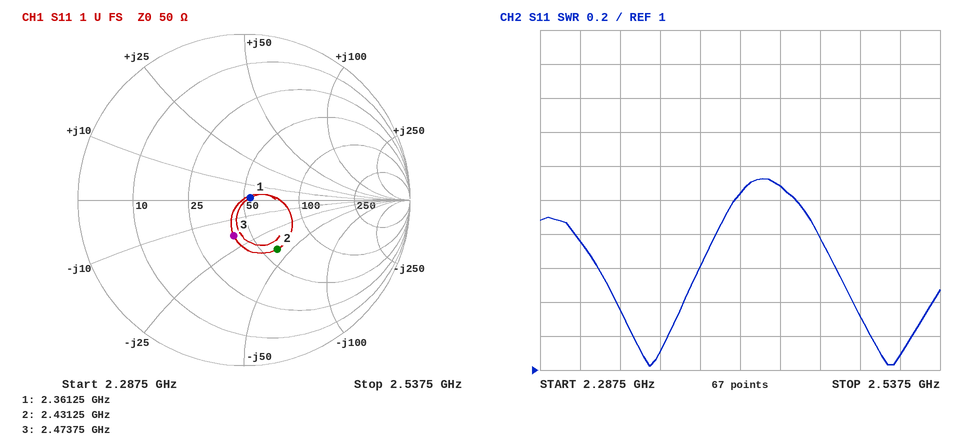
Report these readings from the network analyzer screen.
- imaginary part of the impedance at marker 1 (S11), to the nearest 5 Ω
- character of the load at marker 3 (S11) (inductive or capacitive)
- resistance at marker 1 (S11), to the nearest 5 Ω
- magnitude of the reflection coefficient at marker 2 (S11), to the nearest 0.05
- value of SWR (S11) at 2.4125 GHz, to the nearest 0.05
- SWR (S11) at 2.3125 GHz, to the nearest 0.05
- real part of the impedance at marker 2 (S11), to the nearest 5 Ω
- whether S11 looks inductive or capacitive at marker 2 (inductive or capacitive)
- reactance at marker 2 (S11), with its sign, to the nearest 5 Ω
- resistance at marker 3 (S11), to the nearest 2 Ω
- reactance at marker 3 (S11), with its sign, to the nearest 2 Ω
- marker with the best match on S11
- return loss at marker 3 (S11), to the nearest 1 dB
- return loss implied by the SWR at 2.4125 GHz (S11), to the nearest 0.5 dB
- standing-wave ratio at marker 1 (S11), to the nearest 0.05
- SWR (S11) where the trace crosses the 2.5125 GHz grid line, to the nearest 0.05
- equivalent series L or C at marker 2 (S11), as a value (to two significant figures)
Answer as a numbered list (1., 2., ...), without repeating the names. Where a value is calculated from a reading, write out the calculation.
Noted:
1. 0 Ω
2. capacitive
3. 55 Ω
4. 0.35
5. 2.05
6. 1.75
7. 60 Ω
8. capacitive
9. -40 Ω
10. 40 Ω
11. -18 Ω
12. marker 1
13. 13 dB
14. −20 log10((2.05 − 1)/(2.05 + 1)) ≈ 9.26 dB, so 9.5 dB to the nearest 0.5 dB
15. 1.10
16. 1.10
17. C = 1/(2π × 2.43125 GHz × 40 Ω) ≈ 1.6 pF
